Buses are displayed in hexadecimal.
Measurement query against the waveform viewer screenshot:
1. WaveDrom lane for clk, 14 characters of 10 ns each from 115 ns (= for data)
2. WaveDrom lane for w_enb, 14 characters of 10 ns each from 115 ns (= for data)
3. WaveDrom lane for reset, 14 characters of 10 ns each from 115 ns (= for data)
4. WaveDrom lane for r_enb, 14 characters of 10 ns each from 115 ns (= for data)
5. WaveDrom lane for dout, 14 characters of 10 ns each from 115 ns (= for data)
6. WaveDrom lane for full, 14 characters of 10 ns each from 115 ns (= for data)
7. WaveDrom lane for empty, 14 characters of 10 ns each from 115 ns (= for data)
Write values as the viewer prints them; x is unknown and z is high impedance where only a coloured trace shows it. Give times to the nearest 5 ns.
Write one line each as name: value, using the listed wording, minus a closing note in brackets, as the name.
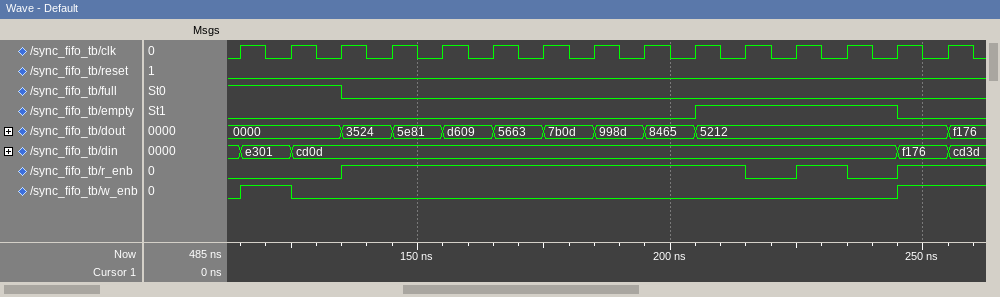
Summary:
WaveDrom lane for clk, 14 characters of 10 ns each from 115 ns: {name: 'clk', wave: 'p.............'}
WaveDrom lane for w_enb, 14 characters of 10 ns each from 115 ns: {name: 'w_enb', wave: '10...........1'}
WaveDrom lane for reset, 14 characters of 10 ns each from 115 ns: {name: 'reset', wave: '0.............'}
WaveDrom lane for r_enb, 14 characters of 10 ns each from 115 ns: {name: 'r_enb', wave: '0.1.......0101'}
WaveDrom lane for dout, 14 characters of 10 ns each from 115 ns: {name: 'dout', wave: '=.========....', data: '0000 3524 5e81 d609 5663 7b0d 998d 8465 5212'}
WaveDrom lane for full, 14 characters of 10 ns each from 115 ns: {name: 'full', wave: '1.0...........'}
WaveDrom lane for empty, 14 characters of 10 ns each from 115 ns: {name: 'empty', wave: '0........1...0'}
